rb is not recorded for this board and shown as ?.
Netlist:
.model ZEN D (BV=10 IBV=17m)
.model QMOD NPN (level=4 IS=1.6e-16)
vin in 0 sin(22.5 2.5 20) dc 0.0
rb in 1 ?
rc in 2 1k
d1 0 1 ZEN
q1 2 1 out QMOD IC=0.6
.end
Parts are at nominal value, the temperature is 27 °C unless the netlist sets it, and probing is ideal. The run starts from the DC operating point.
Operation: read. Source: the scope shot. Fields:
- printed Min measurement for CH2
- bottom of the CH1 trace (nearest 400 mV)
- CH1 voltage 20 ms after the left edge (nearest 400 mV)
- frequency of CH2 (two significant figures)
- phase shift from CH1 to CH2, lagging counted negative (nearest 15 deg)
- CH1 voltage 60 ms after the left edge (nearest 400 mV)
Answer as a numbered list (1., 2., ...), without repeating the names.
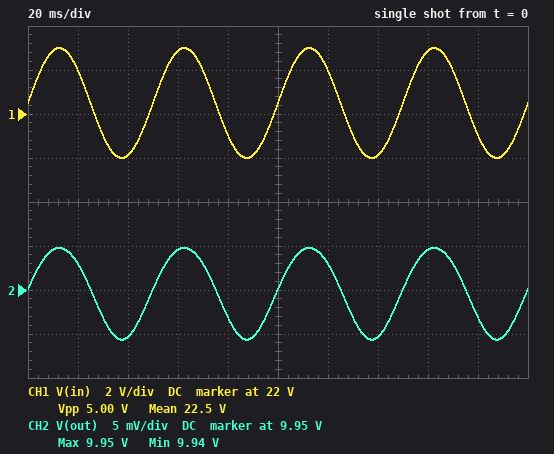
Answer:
1. 9.94 V
2. 20.0 V
3. 24.0 V
4. 20 Hz
5. 0 deg
6. 24.8 V
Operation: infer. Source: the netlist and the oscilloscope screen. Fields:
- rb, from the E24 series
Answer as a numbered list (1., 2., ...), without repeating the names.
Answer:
1. 5.1 kΩ
